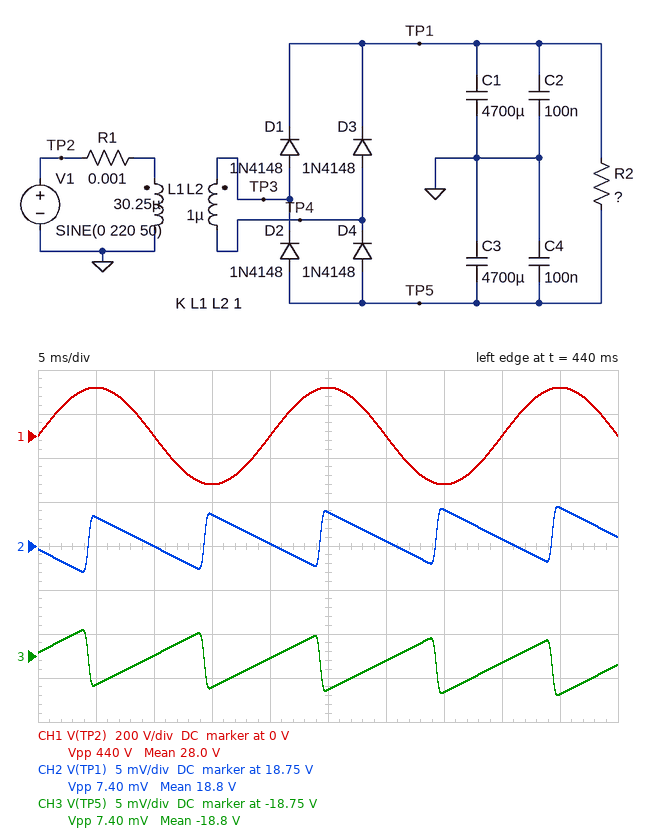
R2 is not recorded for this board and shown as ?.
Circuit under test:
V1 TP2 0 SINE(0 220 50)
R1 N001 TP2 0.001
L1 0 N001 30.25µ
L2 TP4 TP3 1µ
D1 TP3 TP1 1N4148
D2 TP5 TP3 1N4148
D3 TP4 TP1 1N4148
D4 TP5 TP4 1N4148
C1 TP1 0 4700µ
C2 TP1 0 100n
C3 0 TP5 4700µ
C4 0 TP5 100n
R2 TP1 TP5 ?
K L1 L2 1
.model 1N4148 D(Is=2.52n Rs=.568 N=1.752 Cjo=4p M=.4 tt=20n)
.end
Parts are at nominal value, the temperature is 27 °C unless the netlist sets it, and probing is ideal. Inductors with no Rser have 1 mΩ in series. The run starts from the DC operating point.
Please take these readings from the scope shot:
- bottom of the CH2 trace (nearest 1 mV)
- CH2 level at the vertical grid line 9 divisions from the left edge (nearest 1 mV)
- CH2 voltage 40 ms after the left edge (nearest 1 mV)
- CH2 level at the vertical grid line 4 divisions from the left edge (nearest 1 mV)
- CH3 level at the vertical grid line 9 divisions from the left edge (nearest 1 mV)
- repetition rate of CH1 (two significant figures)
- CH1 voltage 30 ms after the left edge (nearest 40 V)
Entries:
18.752 V
18.759 V
18.756 V
18.755 V
-18.759 V
50 Hz
0 V
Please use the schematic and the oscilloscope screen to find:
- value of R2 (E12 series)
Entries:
12 kΩ
